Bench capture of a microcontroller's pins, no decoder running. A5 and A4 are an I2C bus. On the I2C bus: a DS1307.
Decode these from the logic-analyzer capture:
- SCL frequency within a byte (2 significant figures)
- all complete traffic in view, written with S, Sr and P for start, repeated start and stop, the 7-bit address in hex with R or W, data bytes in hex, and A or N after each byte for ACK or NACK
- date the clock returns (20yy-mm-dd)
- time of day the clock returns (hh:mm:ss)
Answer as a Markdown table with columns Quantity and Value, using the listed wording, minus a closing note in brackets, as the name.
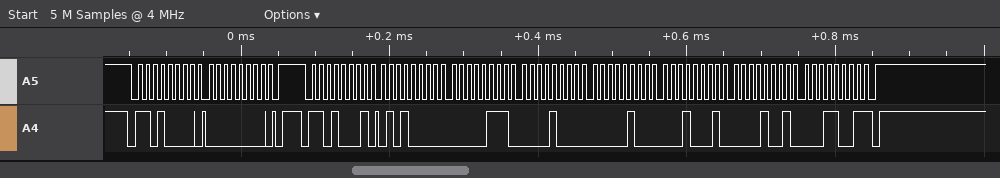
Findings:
| Quantity | Value |
|---|---|
| SCL frequency within a byte | 100 kHz |
| all complete traffic in view, written with S, Sr and P for start, repeated start and stop, the 7-bit address in hex with R or W, data bytes in hex, and A or N after each byte for ACK or NACK | S 68W A 00 A P S 68R A 50 A 07 A 08 A 04 A 11 A 09 A 19 N P |
| date the clock returns | 2019-09-11 |
| time of day the clock returns | 08:07:50 |
